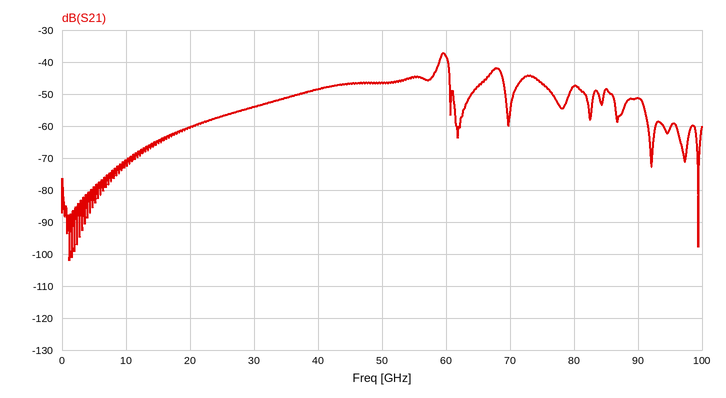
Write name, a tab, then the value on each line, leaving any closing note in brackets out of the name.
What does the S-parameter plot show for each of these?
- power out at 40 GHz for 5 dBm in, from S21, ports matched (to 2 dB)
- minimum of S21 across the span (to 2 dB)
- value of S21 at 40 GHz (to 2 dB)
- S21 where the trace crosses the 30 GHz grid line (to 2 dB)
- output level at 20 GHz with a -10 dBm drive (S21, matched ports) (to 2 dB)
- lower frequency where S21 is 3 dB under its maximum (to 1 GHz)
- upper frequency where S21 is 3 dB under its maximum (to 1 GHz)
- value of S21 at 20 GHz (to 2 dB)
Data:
power out at 40 GHz for 5 dBm in, from S21, ports matched	-44 dBm
minimum of S21 across the span	-102 dB
value of S21 at 40 GHz	-48 dB
S21 where the trace crosses the 30 GHz grid line	-54 dB
output level at 20 GHz with a -10 dBm drive (S21, matched ports)	-70 dBm
lower frequency where S21 is 3 dB under its maximum	59 GHz
upper frequency where S21 is 3 dB under its maximum	60 GHz
value of S21 at 20 GHz	-60 dB
